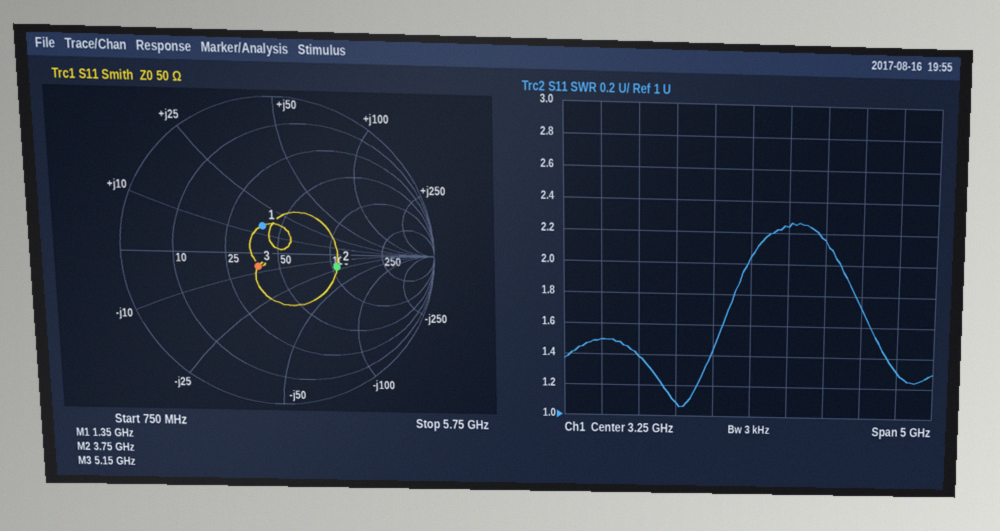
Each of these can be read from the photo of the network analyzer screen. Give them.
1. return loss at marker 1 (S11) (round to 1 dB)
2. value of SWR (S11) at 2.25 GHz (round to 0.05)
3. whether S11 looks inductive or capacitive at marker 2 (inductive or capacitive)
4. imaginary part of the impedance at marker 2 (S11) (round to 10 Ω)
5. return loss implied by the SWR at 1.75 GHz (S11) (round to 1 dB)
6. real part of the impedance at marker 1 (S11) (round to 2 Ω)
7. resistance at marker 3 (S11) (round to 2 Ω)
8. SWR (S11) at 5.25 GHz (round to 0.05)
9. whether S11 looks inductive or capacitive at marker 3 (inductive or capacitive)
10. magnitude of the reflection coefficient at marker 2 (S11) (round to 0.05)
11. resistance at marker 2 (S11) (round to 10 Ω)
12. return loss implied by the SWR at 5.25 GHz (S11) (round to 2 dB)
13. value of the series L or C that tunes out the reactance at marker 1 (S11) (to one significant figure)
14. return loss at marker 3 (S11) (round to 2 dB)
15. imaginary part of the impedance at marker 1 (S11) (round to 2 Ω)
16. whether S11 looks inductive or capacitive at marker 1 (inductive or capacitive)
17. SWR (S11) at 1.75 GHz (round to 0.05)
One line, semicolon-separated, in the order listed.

14 dB; 1.10; capacitive; -20 Ω; 16 dB; 40 Ω; 38 Ω; 1.30; capacitive; 0.40; 110 Ω; 18 dB; 8 pF; 16 dB; +14 Ω; inductive; 1.40
